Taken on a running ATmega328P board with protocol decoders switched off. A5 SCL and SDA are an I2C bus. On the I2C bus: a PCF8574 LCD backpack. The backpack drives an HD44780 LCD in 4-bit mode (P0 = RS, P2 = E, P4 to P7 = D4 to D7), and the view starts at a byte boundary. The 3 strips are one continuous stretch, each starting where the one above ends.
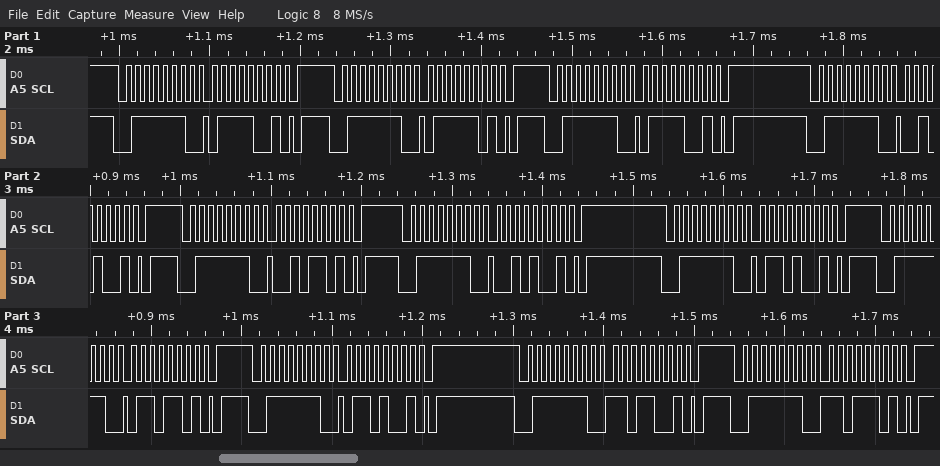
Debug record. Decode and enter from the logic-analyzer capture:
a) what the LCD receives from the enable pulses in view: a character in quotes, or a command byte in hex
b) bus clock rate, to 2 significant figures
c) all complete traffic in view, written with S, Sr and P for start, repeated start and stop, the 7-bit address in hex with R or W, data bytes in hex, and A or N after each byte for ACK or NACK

'r'
100 kHz
S 3FW A 79 A P S 3FW A 7D A P S 3FW A 79 A P S 3FW A 29 A P S 3FW A 2D A P S 3FW A 29 A P S 3FW A 69 A P S 3FW A 6D A P S 3FW A 69 A P S 3FW A D9 A P S 3FW A DD A P
